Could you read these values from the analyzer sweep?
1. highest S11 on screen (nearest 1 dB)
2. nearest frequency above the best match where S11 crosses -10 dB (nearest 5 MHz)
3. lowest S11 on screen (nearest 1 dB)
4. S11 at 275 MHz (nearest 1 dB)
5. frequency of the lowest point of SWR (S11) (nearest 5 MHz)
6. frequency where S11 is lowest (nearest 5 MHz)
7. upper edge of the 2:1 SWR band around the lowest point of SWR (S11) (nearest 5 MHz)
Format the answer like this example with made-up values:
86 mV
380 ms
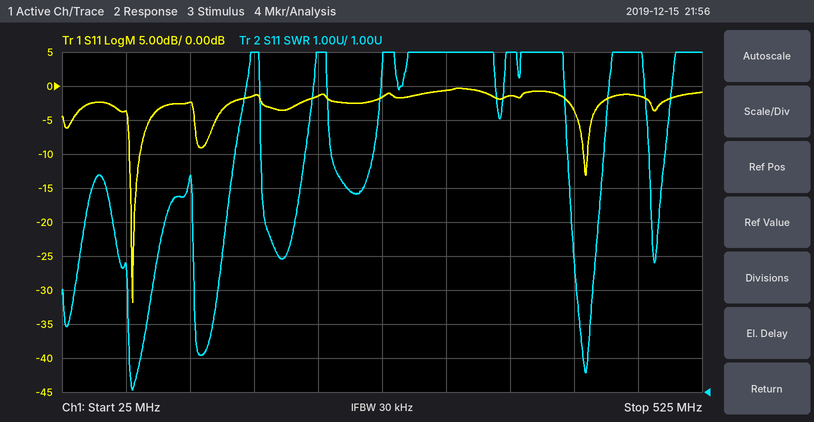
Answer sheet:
0 dB
85 MHz
-32 dB
-2 dB
80 MHz
80 MHz
85 MHz
